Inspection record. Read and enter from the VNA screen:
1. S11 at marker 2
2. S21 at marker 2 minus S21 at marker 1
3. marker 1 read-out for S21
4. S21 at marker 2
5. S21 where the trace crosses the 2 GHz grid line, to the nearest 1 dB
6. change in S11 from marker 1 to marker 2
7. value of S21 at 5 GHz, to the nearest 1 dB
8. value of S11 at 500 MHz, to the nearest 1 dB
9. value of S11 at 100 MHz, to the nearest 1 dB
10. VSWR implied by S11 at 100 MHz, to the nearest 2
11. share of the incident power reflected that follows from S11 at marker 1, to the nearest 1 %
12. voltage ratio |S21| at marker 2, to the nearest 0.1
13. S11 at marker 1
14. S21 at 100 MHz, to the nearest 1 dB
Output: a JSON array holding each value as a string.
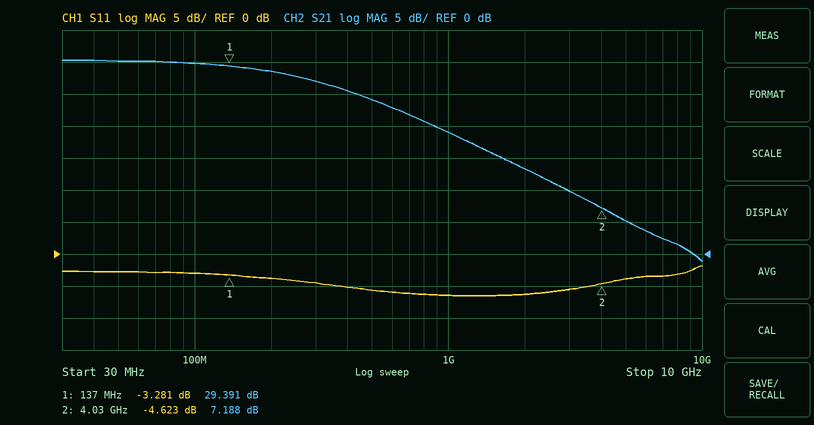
["-4.623 dB", "-22.203 dB", "29.391 dB", "7.188 dB", "13 dB", "-1.342 dB", "5 dB", "-6 dB", "-3 dB", "6", "47 %", "2.3", "-3.281 dB", "30 dB"]
